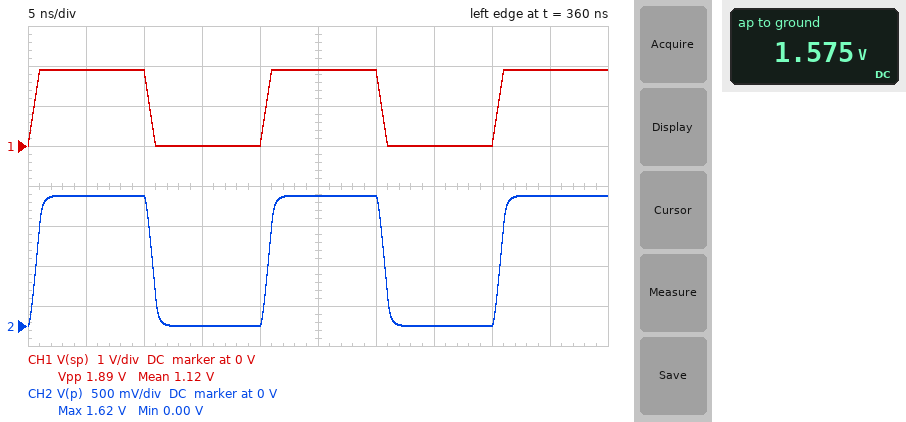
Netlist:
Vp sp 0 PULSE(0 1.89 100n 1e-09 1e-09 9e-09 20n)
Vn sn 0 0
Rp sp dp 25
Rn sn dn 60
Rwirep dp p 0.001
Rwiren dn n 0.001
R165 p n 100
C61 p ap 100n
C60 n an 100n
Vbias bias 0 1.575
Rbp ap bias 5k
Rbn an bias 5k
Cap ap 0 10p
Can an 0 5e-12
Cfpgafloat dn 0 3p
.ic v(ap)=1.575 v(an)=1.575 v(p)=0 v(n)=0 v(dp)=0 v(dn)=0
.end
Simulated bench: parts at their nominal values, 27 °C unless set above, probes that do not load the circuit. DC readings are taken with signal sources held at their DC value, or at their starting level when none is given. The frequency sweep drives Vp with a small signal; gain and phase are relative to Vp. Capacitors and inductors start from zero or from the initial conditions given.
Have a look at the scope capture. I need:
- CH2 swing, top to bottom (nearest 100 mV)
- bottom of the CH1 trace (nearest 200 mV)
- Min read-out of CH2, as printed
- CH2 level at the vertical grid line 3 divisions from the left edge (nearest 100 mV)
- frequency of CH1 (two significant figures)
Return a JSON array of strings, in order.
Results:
["1.6 V", "0 V", "0.00 V", "0 V", "50 MHz"]
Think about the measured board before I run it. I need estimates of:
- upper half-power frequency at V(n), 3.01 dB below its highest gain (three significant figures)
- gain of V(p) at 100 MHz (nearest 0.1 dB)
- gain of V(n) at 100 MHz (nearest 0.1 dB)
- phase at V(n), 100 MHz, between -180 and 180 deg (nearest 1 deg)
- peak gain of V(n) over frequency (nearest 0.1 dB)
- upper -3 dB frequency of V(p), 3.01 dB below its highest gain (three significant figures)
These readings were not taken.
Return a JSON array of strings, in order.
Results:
["373 MHz", "-1.4 dB", "-10.2 dB", "-19 deg", "-9.9 dB", "673 MHz"]
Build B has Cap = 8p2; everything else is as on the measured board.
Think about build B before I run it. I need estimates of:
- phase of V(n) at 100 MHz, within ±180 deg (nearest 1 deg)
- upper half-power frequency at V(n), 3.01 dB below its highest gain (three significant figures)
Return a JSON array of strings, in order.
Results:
["-18 deg", "398 MHz"]
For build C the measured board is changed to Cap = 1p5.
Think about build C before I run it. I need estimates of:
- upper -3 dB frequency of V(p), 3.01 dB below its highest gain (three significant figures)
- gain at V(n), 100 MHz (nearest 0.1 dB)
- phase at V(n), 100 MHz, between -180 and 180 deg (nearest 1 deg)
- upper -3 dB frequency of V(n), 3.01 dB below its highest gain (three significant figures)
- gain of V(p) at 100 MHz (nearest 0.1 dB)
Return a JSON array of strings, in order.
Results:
["4.46 GHz", "-10.1 dB", "-13 deg", "487 MHz", "-1.3 dB"]
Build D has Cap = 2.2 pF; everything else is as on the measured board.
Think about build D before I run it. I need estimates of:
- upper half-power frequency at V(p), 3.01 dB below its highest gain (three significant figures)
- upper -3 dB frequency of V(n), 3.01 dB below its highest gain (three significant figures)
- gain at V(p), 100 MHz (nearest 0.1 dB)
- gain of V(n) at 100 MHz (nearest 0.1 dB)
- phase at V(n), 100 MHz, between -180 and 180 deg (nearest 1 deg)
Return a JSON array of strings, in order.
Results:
["3.03 GHz", "480 MHz", "-1.3 dB", "-10.1 dB", "-13 deg"]
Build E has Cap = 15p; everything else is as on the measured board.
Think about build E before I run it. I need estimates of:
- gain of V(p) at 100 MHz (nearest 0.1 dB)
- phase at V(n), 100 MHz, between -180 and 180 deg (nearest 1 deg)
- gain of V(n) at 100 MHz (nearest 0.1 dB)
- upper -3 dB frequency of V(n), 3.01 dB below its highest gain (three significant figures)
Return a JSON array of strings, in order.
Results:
["-1.5 dB", "-23 deg", "-10.3 dB", "313 MHz"]
